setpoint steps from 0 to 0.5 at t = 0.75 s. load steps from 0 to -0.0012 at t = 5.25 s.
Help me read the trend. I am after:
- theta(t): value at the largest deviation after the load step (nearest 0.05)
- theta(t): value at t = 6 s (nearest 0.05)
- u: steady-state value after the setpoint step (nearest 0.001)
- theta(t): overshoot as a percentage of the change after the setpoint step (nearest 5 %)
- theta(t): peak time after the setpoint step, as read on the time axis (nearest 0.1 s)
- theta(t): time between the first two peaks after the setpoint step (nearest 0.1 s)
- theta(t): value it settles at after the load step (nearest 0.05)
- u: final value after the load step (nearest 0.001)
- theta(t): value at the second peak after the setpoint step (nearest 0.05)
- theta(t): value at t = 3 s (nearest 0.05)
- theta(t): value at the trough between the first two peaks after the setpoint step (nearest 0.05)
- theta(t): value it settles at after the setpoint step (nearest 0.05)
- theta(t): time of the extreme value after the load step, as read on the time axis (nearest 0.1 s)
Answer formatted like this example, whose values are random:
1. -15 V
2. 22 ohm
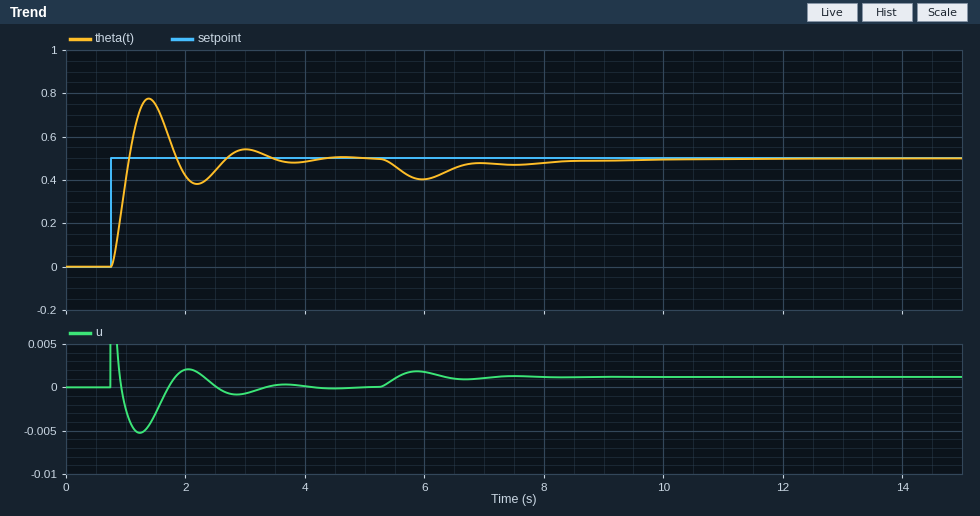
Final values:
1. 0.40
2. 0.40
3. 0.000
4. 55 %
5. 1.4 s
6. 1.6 s
7. 0.50
8. 0.001
9. 0.55
10. 0.55
11. 0.40
12. 0.50
13. 6.0 s
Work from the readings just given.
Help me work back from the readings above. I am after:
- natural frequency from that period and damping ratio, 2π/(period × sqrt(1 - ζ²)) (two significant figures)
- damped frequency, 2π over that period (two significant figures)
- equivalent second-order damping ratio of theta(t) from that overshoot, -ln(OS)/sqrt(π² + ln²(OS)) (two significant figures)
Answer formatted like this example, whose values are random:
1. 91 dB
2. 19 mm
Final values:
1. 4.0 rad/s
2. 3.9 rad/s
3. 0.19
